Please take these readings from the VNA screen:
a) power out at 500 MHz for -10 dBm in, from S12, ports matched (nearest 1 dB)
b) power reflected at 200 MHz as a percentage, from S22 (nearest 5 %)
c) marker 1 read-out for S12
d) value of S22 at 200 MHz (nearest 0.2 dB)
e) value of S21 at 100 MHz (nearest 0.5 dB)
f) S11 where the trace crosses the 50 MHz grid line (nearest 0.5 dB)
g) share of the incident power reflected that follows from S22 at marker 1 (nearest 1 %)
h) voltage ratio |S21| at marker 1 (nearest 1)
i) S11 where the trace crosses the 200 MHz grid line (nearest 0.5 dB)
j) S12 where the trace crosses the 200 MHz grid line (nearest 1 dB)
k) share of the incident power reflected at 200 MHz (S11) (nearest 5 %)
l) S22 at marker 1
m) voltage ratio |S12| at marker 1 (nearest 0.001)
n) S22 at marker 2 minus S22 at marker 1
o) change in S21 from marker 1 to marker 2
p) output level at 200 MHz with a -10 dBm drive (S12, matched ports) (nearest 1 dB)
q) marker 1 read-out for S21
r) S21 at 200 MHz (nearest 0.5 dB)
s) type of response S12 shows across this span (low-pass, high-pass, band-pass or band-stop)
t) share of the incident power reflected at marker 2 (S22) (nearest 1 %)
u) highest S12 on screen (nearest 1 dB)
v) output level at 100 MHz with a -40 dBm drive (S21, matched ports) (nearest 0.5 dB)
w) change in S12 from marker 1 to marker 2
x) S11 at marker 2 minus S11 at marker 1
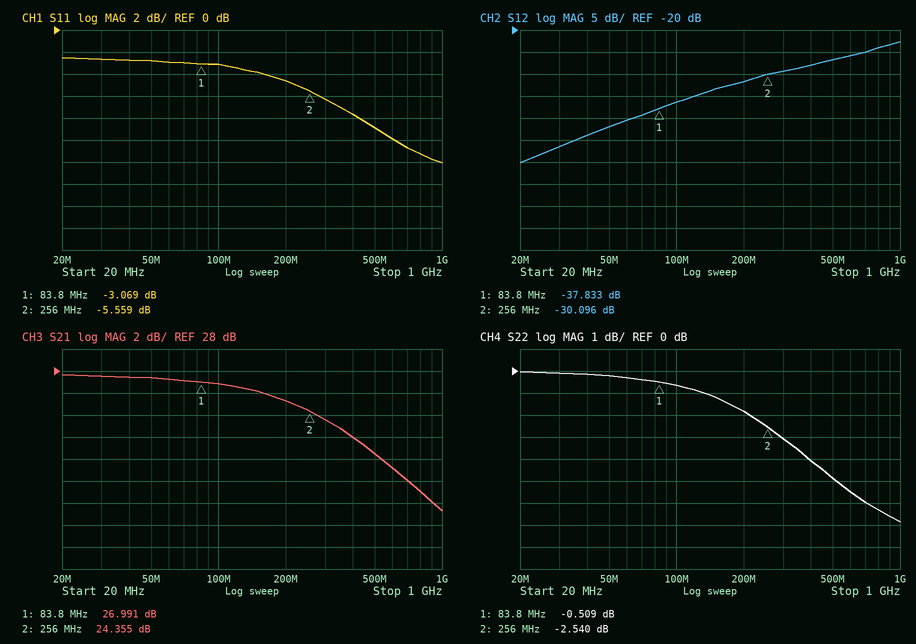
-37 dBm
65 %
-37.833 dB
-1.8 dB
27.0 dB
-3.0 dB
89 %
22
-4.5 dB
-32 dB
35 %
-0.509 dB
0.013
-2.031 dB
-2.636 dB
-42 dBm
26.991 dB
25.5 dB
high-pass
56 %
-23 dB
-13.0 dBm
7.737 dB
-2.490 dB
